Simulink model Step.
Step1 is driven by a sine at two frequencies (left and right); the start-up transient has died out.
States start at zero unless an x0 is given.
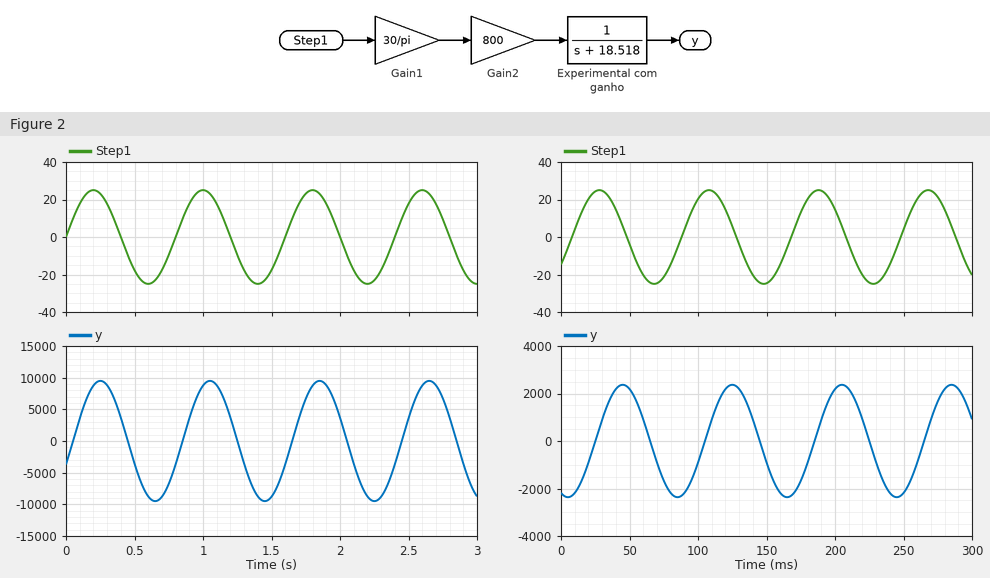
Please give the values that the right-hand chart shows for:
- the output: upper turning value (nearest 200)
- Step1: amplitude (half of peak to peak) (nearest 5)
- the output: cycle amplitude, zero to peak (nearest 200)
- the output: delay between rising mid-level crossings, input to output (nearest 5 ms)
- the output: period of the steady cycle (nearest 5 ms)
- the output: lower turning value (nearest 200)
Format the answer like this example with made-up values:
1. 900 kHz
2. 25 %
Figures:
1. 2400
2. 25
3. 2400
4. 15 ms
5. 80 ms
6. -2400
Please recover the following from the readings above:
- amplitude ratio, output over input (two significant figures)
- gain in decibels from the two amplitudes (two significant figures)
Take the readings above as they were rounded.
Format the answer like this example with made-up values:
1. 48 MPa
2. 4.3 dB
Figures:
1. 96
2. 40 dB
